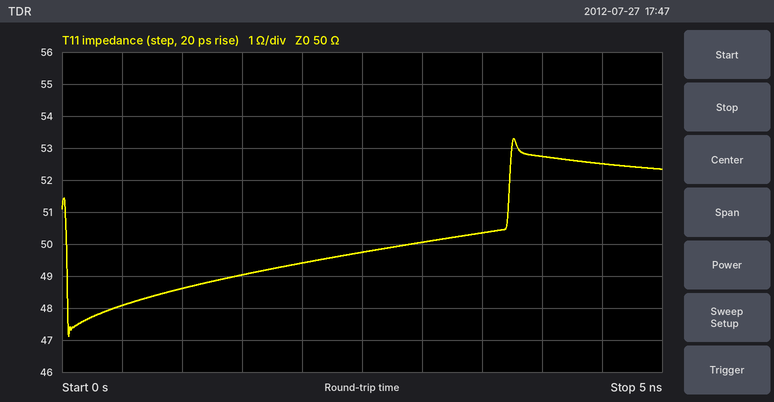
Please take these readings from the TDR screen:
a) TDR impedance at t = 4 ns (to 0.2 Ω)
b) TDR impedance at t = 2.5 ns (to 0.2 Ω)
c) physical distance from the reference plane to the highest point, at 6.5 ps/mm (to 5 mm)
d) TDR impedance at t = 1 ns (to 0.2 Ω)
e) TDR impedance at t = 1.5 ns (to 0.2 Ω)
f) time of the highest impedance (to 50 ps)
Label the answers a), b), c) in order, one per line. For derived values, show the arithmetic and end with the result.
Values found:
a) 52.8 Ω
b) 49.8 Ω
c) 3.75 ns / 2 / 6.5 ps/mm ≈ 288 mm, so 290 mm to the nearest 5 mm
d) 48.6 Ω
e) 49.0 Ω
f) 3.75 ns
